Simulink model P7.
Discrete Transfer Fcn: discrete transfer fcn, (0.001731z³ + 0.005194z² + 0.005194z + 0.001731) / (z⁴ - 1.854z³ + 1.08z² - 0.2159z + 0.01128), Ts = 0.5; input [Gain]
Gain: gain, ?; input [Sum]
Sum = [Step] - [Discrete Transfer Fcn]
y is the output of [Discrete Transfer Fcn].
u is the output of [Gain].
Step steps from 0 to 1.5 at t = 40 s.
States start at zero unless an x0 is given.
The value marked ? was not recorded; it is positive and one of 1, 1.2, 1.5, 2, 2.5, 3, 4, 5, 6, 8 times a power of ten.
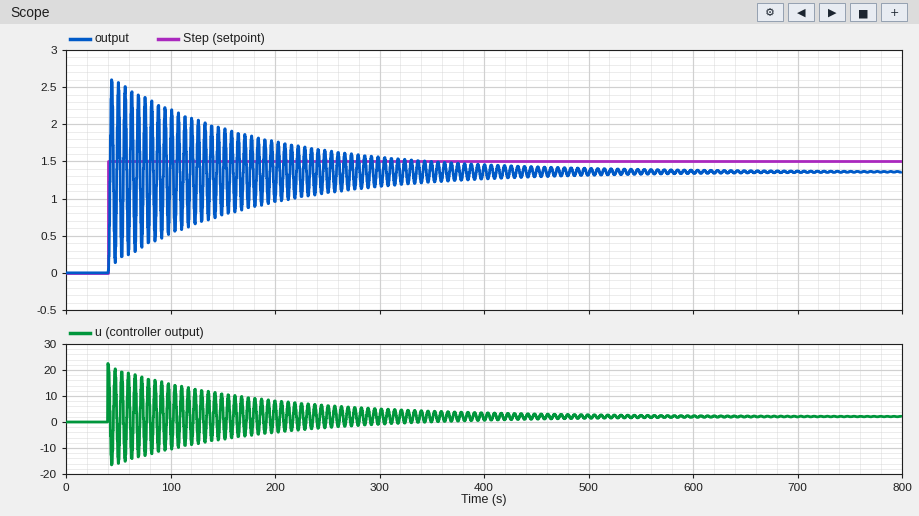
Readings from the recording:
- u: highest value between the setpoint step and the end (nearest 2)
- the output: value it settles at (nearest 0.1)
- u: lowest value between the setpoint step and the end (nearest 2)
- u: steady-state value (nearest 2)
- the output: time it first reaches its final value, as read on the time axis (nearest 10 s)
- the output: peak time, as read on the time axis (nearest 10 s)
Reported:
22
1.4
-16
2
40 s
40 s
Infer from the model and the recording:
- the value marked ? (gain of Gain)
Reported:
15
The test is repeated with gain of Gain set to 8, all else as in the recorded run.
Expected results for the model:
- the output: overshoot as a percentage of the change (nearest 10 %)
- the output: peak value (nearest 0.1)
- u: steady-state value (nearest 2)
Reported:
50 %
1.9
2
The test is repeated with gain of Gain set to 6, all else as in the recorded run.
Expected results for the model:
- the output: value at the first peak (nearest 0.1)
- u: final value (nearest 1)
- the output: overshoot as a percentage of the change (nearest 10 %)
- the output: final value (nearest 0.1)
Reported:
1.6
2
30 %
1.2
